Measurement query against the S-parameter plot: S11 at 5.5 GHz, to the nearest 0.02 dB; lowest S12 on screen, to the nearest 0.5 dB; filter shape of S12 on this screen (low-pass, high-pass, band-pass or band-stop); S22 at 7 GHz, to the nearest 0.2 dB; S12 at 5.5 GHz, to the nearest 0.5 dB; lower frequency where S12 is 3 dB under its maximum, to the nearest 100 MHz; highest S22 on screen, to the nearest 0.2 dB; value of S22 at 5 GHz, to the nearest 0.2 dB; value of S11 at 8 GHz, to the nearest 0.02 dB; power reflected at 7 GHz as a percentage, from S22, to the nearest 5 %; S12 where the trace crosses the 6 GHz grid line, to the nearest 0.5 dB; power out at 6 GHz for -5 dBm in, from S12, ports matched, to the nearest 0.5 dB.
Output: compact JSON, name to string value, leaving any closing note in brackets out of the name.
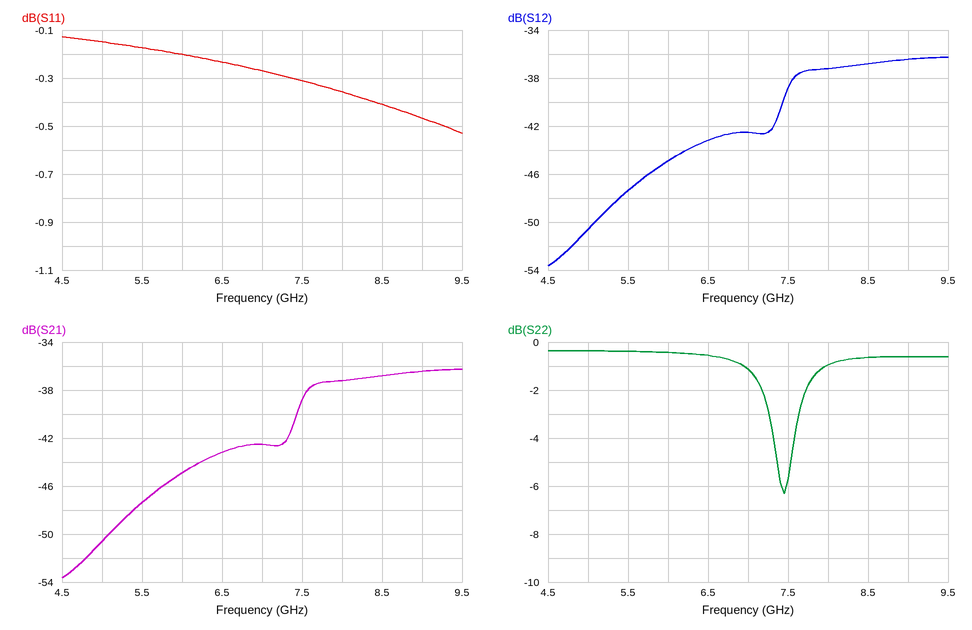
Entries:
{"S11 at 5.5 GHz, to the nearest 0.02 dB": "-0.18 dB", "lowest S12 on screen, to the nearest 0.5 dB": "-53.5 dB", "filter shape of S12 on this screen": "high-pass", "S22 at 7 GHz, to the nearest 0.2 dB": "-1.2 dB", "S12 at 5.5 GHz, to the nearest 0.5 dB": "-47.5 dB", "lower frequency where S12 is 3 dB under its maximum, to the nearest 100 MHz": "7.5 GHz", "highest S22 on screen, to the nearest 0.2 dB": "-0.4 dB", "value of S22 at 5 GHz, to the nearest 0.2 dB": "-0.4 dB", "value of S11 at 8 GHz, to the nearest 0.02 dB": "-0.36 dB", "power reflected at 7 GHz as a percentage, from S22, to the nearest 5 %": "75 %", "S12 where the trace crosses the 6 GHz grid line, to the nearest 0.5 dB": "-45.0 dB", "power out at 6 GHz for -5 dBm in, from S12, ports matched, to the nearest 0.5 dB": "-50.0 dBm"}
